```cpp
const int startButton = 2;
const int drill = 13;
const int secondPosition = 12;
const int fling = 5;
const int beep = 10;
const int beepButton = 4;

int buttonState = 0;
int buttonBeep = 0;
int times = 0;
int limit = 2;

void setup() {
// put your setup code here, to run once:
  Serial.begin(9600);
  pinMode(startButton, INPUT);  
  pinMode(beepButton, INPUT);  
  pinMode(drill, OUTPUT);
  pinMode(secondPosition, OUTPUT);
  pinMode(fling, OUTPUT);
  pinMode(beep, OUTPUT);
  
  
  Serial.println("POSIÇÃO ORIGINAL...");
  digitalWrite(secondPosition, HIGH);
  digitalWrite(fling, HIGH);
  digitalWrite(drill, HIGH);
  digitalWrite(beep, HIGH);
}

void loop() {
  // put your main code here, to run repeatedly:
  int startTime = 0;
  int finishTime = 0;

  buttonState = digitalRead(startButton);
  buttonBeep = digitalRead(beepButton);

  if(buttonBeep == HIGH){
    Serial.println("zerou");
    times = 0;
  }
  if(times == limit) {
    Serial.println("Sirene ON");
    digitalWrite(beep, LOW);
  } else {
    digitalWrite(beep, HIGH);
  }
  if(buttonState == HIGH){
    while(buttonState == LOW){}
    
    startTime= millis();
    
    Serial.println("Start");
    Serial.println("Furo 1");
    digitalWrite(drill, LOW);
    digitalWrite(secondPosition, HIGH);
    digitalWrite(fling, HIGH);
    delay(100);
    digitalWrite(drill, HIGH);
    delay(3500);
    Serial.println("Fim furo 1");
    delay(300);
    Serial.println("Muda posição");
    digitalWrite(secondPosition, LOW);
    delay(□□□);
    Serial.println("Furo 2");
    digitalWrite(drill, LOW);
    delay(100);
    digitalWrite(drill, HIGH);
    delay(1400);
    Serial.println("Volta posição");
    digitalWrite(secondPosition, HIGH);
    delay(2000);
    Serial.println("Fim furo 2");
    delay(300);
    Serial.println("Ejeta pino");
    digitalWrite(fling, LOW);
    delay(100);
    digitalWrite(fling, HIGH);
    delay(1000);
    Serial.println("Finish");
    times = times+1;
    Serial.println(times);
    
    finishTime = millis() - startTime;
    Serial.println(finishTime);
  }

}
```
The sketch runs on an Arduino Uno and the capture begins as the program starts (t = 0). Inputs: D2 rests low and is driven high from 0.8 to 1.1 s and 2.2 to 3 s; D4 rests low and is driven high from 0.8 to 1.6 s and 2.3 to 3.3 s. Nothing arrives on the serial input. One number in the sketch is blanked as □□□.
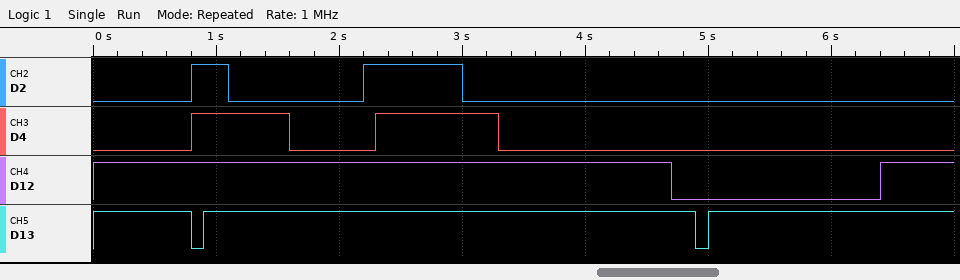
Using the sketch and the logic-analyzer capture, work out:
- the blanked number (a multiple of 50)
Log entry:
200
